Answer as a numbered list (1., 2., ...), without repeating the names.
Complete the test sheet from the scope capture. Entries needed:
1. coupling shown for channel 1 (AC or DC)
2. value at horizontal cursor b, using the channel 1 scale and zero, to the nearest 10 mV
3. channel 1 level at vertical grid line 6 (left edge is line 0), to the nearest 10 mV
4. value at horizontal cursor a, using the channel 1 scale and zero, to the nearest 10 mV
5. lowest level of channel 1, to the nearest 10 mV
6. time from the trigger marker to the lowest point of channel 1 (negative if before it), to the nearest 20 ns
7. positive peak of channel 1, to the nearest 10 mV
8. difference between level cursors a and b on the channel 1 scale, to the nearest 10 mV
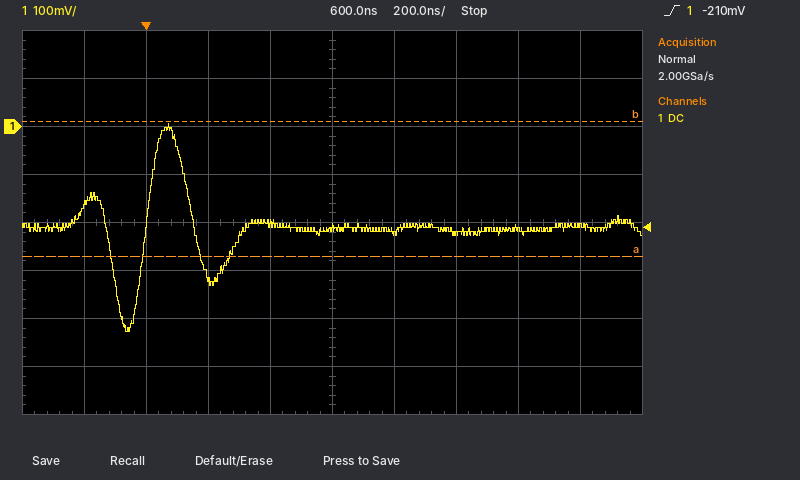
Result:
1. DC
2. 10 mV
3. -220 mV
4. -270 mV
5. -430 mV
6. -60 ns
7. 10 mV
8. 280 mV
